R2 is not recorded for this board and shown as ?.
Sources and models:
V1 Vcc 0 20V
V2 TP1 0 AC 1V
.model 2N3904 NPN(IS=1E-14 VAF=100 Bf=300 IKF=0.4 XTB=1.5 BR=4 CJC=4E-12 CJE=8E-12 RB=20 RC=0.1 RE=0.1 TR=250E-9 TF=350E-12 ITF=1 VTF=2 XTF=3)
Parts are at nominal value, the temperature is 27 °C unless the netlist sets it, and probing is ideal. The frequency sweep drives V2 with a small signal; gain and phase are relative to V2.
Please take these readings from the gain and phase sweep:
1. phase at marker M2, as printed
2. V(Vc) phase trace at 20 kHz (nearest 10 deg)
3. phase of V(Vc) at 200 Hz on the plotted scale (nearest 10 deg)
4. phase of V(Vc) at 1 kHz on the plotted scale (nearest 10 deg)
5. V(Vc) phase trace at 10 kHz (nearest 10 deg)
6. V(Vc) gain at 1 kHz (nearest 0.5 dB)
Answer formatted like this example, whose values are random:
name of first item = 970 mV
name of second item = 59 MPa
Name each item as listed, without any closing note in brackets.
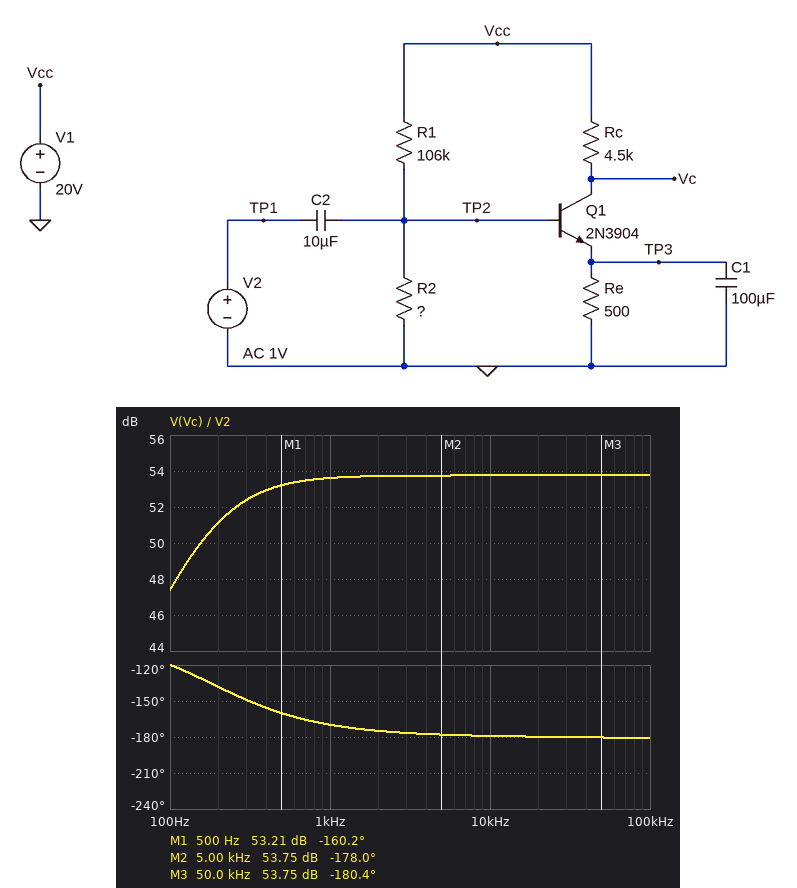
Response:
phase at marker M2, as printed = -178.0 deg
V(Vc) phase trace at 20 kHz = -180 deg
phase of V(Vc) at 200 Hz on the plotted scale = -140 deg
phase of V(Vc) at 1 kHz on the plotted scale = -170 deg
V(Vc) phase trace at 10 kHz = -180 deg
V(Vc) gain at 1 kHz = 53.5 dB
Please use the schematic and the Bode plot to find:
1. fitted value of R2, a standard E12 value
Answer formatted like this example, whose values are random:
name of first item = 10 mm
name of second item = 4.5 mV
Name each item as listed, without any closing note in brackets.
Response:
fitted value of R2, a standard E12 value = 15 kΩ
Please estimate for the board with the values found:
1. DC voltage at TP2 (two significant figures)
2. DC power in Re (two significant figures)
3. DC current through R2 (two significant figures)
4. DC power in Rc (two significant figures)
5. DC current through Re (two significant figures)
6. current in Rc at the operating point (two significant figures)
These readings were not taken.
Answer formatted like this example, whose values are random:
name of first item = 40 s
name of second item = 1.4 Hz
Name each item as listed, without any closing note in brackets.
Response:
DC voltage at TP2 = 2.3 V
DC power in Re = 5.5 mW
DC current through R2 = 160 µA
DC power in Rc = 49 mW
DC current through Re = 3.3 mA
current in Rc at the operating point = 3.3 mA
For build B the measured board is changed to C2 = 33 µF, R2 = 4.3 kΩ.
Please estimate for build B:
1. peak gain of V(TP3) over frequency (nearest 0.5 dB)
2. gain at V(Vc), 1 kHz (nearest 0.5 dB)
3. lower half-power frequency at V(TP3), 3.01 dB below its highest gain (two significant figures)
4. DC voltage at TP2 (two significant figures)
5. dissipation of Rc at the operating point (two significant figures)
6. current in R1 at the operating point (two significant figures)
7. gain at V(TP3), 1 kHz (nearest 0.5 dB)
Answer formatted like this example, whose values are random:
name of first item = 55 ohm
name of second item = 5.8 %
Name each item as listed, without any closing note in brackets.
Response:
peak gain of V(TP3) over frequency = -2.0 dB
gain at V(Vc), 1 kHz = 34.5 dB
lower half-power frequency at V(TP3), 3.01 dB below its highest gain = 1.1 Hz
DC voltage at TP2 = 780 mV
dissipation of Rc at the operating point = 430 µW
current in R1 at the operating point = 180 µA
gain at V(TP3), 1 kHz = -34.5 dB
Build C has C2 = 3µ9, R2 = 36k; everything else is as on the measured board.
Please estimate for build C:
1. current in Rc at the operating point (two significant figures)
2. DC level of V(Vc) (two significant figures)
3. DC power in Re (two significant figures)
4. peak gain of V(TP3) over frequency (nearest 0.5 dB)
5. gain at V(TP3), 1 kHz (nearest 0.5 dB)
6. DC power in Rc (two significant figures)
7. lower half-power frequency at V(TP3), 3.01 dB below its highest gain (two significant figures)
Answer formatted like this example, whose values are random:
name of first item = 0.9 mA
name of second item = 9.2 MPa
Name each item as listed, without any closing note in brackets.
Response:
current in Rc at the operating point = 4.0 mA
DC level of V(Vc) = 2.1 V
DC power in Re = 8.3 mW
peak gain of V(TP3) over frequency = -28.0 dB
gain at V(TP3), 1 kHz = -31.5 dB
DC power in Rc = 71 mW
lower half-power frequency at V(TP3), 3.01 dB below its highest gain = 3.4 Hz
